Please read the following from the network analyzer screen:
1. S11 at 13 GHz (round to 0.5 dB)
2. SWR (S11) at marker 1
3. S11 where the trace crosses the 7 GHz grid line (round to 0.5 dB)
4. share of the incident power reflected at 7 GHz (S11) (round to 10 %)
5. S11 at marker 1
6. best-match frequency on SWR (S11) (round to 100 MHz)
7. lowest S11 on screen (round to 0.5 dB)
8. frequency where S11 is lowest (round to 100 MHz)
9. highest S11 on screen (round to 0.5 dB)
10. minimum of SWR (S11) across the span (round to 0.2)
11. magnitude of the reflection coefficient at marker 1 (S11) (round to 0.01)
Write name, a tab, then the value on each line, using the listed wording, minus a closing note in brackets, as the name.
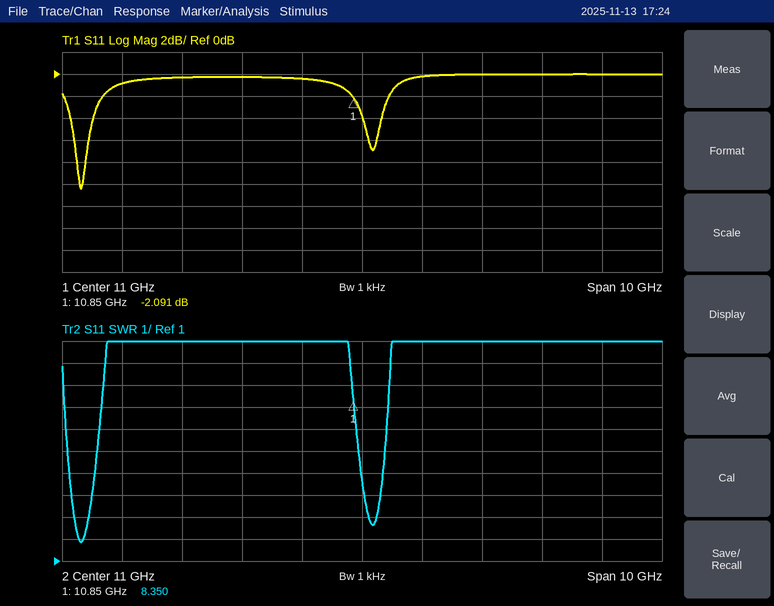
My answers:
S11 at 13 GHz	0.0 dB
SWR (S11) at marker 1	8.350
S11 where the trace crosses the 7 GHz grid line	-1.0 dB
share of the incident power reflected at 7 GHz (S11)	80 %
S11 at marker 1	-2.091 dB
best-match frequency on SWR (S11)	6.3 GHz
lowest S11 on screen	-10.5 dB
frequency where S11 is lowest	6.3 GHz
highest S11 on screen	0.0 dB
minimum of SWR (S11) across the span	1.8
magnitude of the reflection coefficient at marker 1 (S11)	0.79
